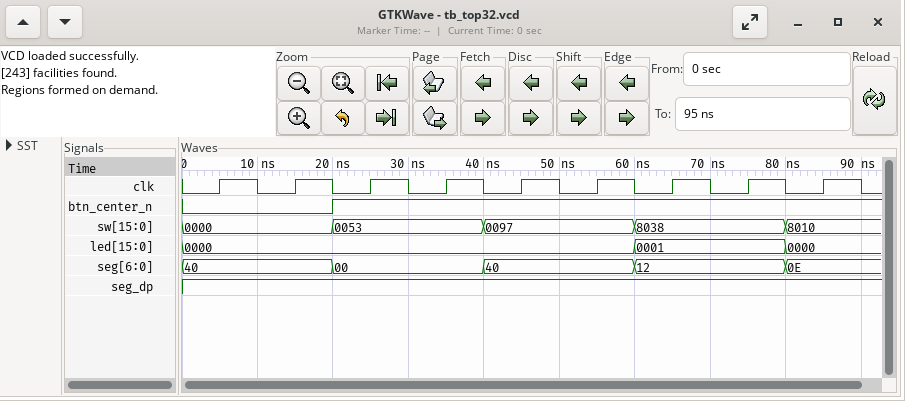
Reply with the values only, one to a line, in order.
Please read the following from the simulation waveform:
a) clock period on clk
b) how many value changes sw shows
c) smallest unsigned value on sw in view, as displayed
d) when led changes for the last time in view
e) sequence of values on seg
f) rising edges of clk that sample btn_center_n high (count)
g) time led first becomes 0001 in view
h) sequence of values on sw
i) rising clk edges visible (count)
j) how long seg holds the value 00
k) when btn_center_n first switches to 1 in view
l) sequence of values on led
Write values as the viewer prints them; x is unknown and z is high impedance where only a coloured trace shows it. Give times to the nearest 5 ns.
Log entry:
10 ns
4
0000
80 ns
40, 00, 40, 12, 0E
7
60 ns
0000, 0053, 0097, 8038, 8010
9
20 ns
20 ns
0000, 0001, 0000
